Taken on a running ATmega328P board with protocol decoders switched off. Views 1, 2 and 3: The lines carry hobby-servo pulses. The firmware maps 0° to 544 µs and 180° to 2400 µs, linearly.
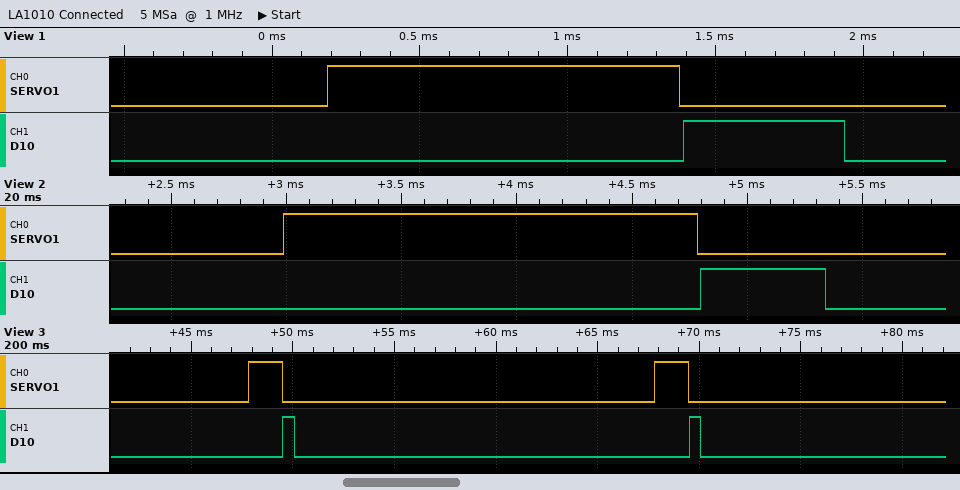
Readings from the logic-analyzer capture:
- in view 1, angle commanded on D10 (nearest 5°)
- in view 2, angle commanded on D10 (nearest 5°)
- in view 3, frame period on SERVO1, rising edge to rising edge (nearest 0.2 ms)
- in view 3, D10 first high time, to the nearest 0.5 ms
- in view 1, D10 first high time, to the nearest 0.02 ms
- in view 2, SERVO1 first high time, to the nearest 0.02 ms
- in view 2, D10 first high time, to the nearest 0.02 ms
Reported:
0°
0°
20.0 ms
0.5 ms
0.54 ms
1.80 ms
0.54 ms
